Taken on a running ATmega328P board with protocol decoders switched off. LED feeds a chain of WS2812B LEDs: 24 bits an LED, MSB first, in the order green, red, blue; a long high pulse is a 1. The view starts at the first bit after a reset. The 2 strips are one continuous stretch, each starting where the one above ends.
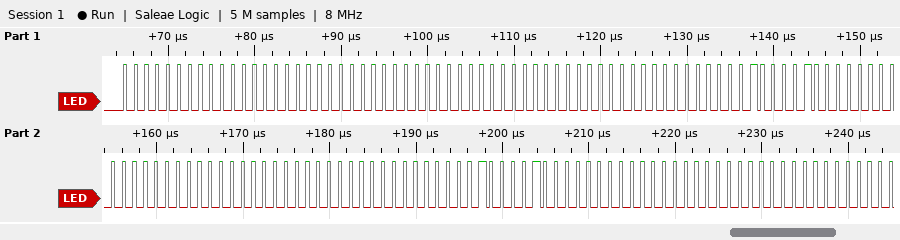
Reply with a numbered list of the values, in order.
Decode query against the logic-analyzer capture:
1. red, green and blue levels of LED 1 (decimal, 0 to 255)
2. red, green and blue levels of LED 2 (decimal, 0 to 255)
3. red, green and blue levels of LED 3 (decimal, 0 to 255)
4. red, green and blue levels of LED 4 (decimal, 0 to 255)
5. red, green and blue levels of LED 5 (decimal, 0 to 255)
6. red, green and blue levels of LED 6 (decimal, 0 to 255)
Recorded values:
1. 0, 0, 0
2. 0, 0, 0
3. 33, 0, 0
4. 0, 0, 0
5. 33, 0, 0
6. 0, 0, 0
